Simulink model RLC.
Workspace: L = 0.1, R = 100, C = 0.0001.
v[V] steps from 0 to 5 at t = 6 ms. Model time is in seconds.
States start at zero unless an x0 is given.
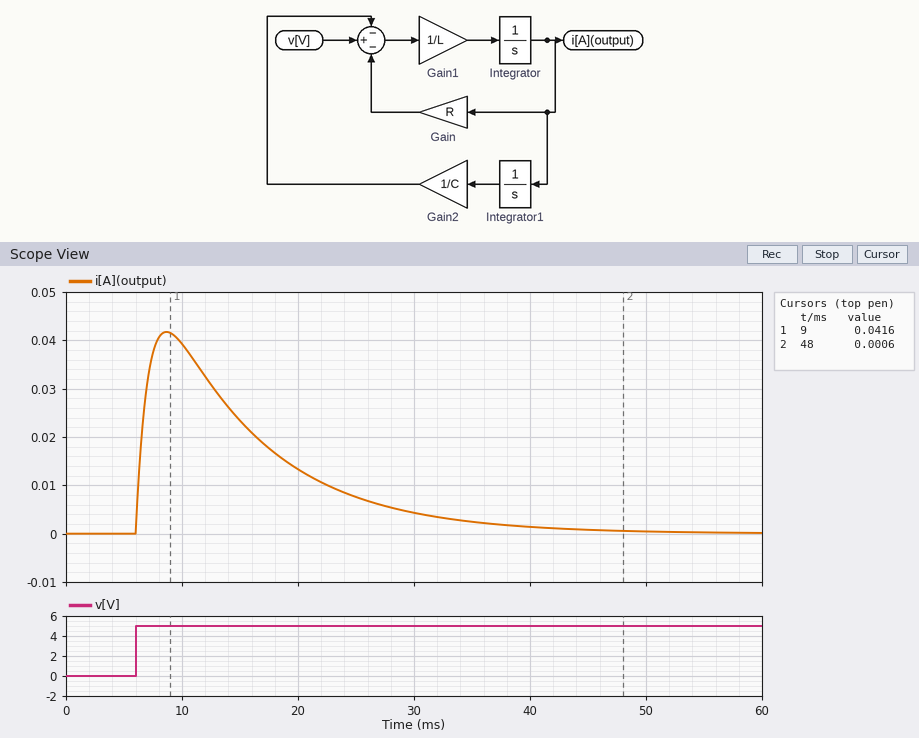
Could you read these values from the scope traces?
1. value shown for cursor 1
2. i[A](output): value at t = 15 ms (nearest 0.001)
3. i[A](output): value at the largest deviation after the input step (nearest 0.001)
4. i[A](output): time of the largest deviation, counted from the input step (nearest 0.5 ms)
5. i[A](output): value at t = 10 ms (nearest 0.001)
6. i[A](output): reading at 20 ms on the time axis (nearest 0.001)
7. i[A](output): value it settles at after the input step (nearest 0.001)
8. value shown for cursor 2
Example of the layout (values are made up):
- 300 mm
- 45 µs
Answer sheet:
- 0.0416
- 0.023
- 0.042
- 2.5 ms
- 0.039
- 0.013
- 0.000
- 0.0006
